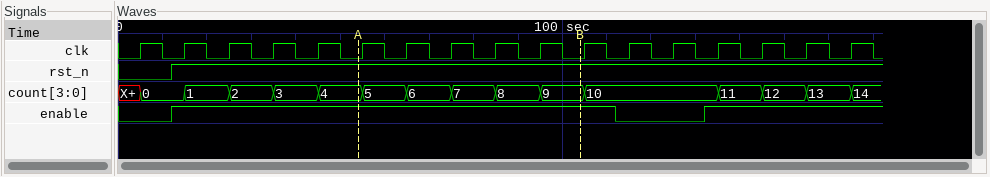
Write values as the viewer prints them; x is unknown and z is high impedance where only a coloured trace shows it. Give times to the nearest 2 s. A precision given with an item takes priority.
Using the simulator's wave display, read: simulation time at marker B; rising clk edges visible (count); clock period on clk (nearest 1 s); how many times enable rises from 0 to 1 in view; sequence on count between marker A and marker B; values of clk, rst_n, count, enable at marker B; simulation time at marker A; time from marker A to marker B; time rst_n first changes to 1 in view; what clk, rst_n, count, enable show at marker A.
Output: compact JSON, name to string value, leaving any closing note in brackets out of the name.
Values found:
{"simulation time at marker B": "104 s", "rising clk edges visible": "17", "clock period on clk": "10 s", "how many times enable rises from 0 to 1 in view": "2", "sequence on count between marker A and marker B": "4, 5, 6, 7, 8, 9", "values of clk, rst_n, count, enable at marker B": "clk=0, rst_n=1, count=9, enable=1", "simulation time at marker A": "54 s", "time from marker A to marker B": "50 s", "time rst_n first changes to 1 in view": "12 s", "what clk, rst_n, count, enable show at marker A": "clk=0, rst_n=1, count=4, enable=1"}
